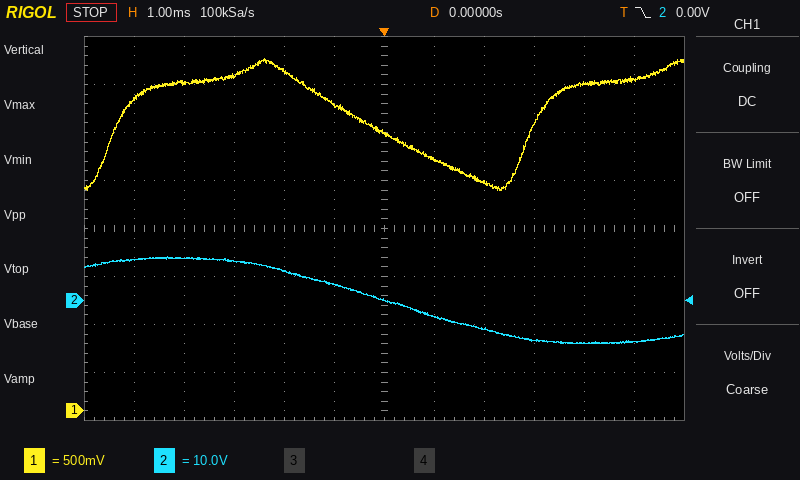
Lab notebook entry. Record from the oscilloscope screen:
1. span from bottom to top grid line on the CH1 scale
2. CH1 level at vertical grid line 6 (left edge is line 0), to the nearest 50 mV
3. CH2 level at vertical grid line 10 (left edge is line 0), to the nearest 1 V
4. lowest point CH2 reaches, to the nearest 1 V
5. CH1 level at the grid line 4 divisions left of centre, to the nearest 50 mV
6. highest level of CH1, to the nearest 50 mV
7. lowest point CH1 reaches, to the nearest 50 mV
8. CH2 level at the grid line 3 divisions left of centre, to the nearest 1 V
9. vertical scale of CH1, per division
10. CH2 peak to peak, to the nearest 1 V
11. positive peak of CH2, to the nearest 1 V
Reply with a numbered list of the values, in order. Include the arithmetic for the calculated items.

1. 4 V
2. 2.90 V
3. -9 V
4. -9 V
5. 3.40 V
6. 3.65 V
7. 2.30 V
8. 8 V
9. 500 mV
10. 9 V − (-9 V) = 18 V
11. 9 V
